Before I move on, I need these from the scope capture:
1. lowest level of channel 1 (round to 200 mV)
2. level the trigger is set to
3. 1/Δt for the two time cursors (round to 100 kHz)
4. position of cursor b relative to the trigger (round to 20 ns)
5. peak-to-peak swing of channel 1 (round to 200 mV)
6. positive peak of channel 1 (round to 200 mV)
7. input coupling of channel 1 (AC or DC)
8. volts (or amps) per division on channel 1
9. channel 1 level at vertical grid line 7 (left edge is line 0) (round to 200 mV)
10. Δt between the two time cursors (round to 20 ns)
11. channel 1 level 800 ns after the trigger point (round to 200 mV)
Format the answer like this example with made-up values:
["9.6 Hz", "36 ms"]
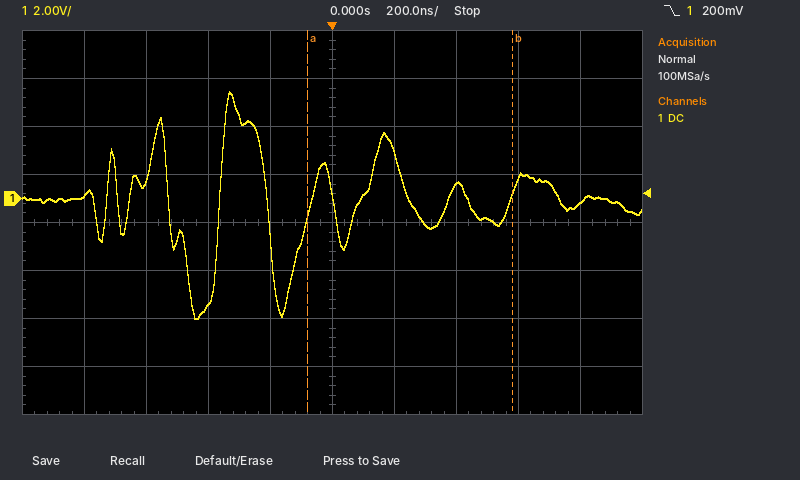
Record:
["-5.0 V", "200 mV", "1.5 MHz", "+580 ns", "9.4 V", "4.4 V", "DC", "2 V", "600 mV", "660 ns", "-200 mV"]
